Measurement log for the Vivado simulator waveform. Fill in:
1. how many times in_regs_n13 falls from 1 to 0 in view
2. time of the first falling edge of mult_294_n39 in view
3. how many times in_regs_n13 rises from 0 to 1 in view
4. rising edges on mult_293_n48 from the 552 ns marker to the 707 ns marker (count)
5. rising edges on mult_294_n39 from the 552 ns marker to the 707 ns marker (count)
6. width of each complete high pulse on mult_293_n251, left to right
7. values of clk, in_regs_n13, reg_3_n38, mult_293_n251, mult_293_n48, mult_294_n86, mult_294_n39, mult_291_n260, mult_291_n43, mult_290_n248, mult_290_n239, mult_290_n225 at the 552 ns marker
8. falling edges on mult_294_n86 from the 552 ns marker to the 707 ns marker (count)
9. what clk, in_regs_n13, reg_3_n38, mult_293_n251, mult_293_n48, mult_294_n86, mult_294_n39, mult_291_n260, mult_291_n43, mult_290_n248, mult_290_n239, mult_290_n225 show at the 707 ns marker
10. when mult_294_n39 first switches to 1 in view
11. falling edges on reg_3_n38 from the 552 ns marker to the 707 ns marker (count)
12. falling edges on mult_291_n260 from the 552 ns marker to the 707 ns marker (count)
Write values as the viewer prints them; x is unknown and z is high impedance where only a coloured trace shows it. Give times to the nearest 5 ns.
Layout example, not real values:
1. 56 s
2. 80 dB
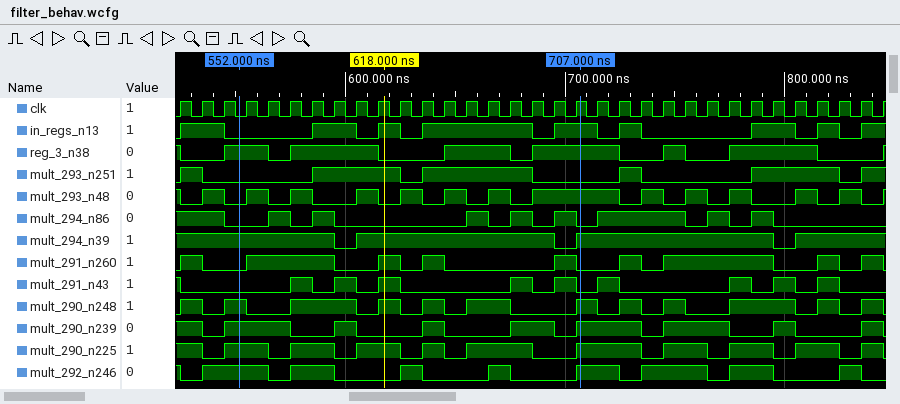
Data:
1. 8
2. 595 ns
3. 9
4. 7
5. 2
6. 10 ns, 40 ns, 50 ns, 10 ns, 40 ns
7. clk=0, in_regs_n13=0, reg_3_n38=1, mult_293_n251=0, mult_293_n48=0, mult_294_n86=0, mult_294_n39=1, mult_291_n260=0, mult_291_n43=0, mult_290_n248=1, mult_290_n239=1, mult_290_n225=1
8. 5
9. clk=1, in_regs_n13=1, reg_3_n38=1, mult_293_n251=0, mult_293_n48=1, mult_294_n86=0, mult_294_n39=1, mult_291_n260=0, mult_291_n43=0, mult_290_n248=1, mult_290_n239=1, mult_290_n225=1
10. 605 ns
11. 3
12. 4
